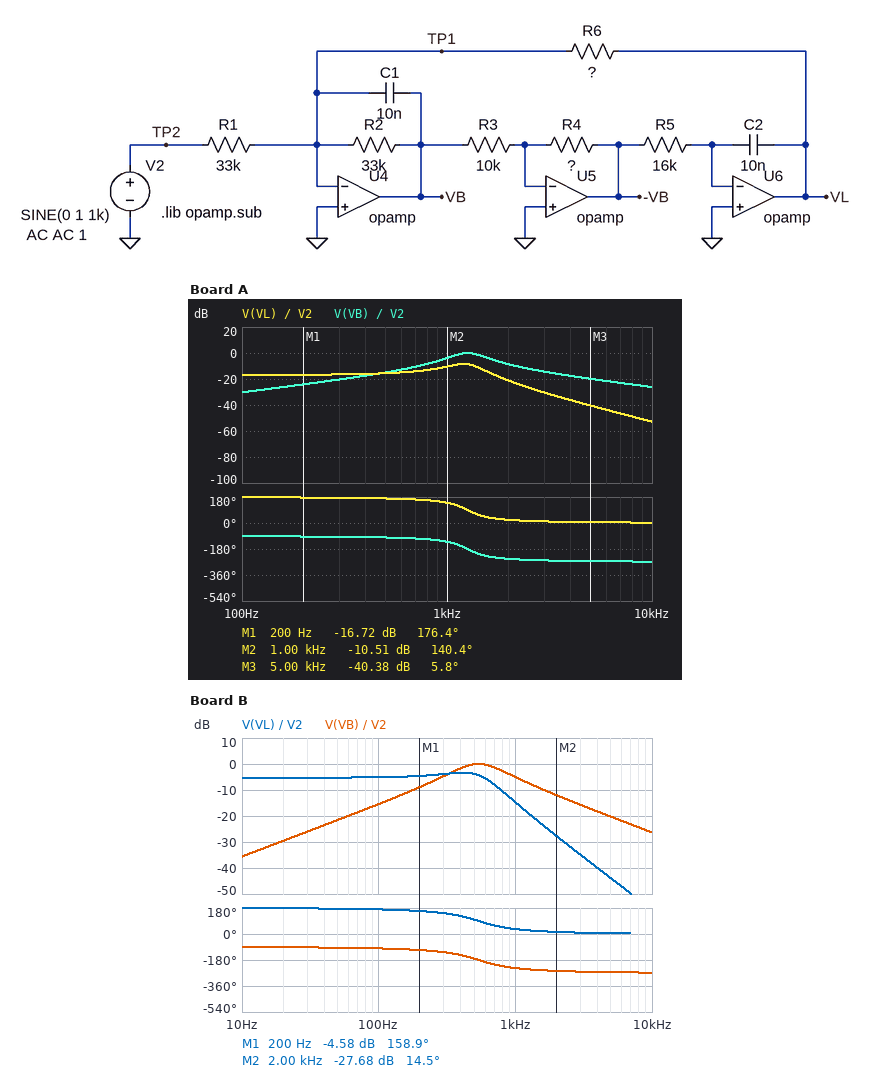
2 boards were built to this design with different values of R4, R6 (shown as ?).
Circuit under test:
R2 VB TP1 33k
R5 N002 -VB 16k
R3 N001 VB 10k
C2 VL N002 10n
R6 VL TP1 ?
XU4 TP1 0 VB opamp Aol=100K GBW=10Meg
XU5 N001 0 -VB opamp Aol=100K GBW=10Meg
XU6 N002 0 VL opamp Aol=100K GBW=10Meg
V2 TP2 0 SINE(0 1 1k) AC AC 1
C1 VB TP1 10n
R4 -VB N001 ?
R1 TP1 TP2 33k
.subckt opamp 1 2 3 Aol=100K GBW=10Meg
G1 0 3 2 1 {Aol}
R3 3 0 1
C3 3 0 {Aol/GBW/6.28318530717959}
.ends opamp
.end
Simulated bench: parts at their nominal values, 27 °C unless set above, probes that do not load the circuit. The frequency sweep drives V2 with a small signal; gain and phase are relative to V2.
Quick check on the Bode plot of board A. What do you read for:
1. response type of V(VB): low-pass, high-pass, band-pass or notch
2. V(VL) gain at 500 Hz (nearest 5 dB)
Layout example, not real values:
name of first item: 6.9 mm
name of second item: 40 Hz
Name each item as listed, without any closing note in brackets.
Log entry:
response type of V(VB): low-pass, high-pass, band-pass or notch: band-pass
V(VL) gain at 500 Hz: -15 dB
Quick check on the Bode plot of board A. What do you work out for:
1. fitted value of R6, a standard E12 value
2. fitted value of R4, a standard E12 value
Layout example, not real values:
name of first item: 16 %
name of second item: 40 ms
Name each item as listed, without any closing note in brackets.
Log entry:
fitted value of R6, a standard E12 value: 4.7 kΩ
fitted value of R4, a standard E12 value: 4.7 kΩ
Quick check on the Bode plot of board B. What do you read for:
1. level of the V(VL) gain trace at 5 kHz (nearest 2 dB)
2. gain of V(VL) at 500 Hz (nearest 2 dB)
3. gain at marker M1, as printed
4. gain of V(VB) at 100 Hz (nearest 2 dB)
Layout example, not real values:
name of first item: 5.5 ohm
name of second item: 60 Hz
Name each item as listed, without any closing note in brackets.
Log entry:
level of the V(VL) gain trace at 5 kHz: -44 dB
gain of V(VL) at 500 Hz: -4 dB
gain at marker M1, as printed: -4.58 dB
gain of V(VB) at 100 Hz: -16 dB
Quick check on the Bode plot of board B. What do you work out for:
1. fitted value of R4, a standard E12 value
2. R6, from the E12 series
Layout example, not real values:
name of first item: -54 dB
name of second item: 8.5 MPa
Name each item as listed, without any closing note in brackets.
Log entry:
fitted value of R4, a standard E12 value: 3.3 kΩ
R6, from the E12 series: 18 kΩ
